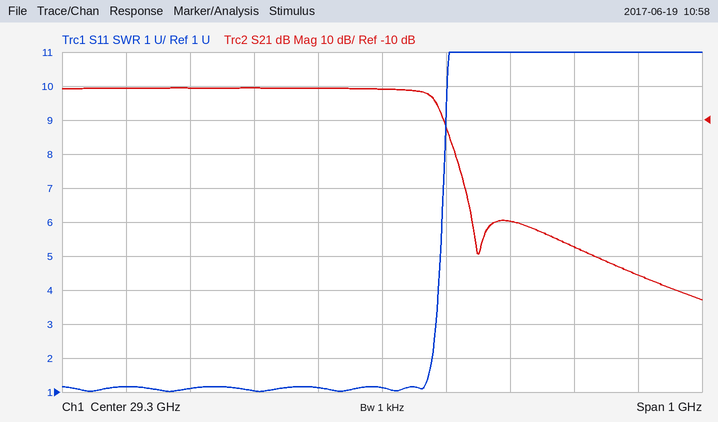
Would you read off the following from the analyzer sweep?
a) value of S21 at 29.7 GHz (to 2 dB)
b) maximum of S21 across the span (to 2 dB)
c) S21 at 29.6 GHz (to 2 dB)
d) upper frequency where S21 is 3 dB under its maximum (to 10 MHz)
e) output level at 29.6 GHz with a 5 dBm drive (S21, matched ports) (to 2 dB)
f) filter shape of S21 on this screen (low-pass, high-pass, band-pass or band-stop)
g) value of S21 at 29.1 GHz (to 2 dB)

-56 dB
0 dB
-48 dB
29.38 GHz
-42 dBm
low-pass
0 dB
